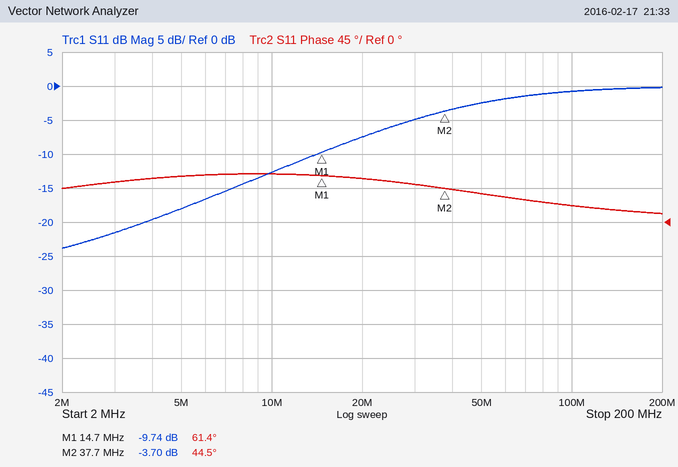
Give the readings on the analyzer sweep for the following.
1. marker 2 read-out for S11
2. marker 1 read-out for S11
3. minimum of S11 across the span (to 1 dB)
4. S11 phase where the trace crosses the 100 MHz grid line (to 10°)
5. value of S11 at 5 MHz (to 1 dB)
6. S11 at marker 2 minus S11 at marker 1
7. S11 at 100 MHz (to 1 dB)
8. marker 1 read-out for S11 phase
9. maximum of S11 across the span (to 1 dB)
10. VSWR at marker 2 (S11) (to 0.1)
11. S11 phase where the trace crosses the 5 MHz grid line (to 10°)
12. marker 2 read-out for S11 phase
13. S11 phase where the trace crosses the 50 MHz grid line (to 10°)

-3.70 dB
-9.74 dB
-24 dB
20°
-18 dB
6.04 dB
-1 dB
61.4°
0 dB
4.8
60°
44.5°
40°
